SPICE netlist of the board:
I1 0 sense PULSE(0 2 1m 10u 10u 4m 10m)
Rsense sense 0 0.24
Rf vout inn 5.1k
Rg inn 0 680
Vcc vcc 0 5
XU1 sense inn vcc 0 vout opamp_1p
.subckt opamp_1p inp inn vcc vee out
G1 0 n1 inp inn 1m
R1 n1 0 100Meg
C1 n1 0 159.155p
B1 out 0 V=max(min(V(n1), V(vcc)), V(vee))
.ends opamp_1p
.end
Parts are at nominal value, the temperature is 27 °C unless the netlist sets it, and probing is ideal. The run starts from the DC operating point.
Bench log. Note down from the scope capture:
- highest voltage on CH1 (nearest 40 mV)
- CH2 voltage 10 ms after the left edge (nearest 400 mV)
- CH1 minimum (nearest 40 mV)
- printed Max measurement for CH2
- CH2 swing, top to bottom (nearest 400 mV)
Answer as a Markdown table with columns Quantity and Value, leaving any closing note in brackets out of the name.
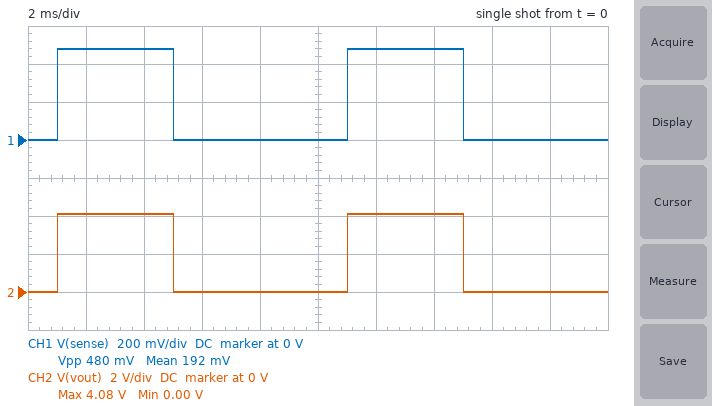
| Quantity | Value |
|---|---|
| highest voltage on CH1 | 480 mV |
| CH2 voltage 10 ms after the left edge | 0 V |
| CH1 minimum | 0 V |
| printed Max measurement for CH2 | 4.08 V |
| CH2 swing, top to bottom | 4.0 V |
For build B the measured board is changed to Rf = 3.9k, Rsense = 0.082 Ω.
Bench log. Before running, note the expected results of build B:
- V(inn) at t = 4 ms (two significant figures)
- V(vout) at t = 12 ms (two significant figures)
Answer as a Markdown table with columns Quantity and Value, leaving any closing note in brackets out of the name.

| Quantity | Value |
|---|---|
| V(inn) at t = 4 ms | 160 mV |
| V(vout) at t = 12 ms | 1.1 V |
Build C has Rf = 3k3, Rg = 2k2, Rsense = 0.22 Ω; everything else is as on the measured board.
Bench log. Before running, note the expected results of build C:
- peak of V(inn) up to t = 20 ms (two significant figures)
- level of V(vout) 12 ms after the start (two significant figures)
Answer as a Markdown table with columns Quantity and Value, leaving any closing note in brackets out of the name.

| Quantity | Value |
|---|---|
| peak of V(inn) up to t = 20 ms | 440 mV |
| level of V(vout) 12 ms after the start | 1.1 V |
